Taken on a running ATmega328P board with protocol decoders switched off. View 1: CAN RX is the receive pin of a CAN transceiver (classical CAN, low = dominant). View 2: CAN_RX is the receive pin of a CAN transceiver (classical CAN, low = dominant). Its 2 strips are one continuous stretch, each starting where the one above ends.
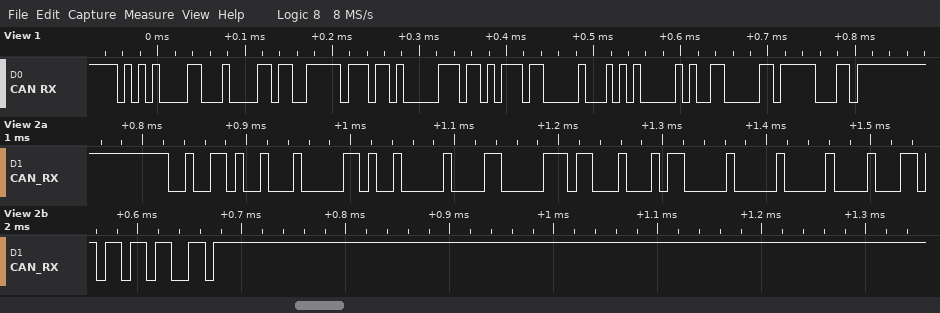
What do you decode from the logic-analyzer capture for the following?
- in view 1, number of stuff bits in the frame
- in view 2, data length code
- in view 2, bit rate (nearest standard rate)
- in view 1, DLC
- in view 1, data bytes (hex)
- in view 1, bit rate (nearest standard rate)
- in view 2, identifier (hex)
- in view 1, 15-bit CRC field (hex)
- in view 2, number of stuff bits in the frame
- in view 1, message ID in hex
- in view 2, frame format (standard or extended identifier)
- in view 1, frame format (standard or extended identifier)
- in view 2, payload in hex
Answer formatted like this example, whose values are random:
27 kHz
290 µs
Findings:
6
8
125 kbit/s
8
6C FF 68 36 BB 00 A8 13
125 kbit/s
0x269
0x02F9
6
0x543
standard
standard
29 00 60 D8 8B 00 00 11
